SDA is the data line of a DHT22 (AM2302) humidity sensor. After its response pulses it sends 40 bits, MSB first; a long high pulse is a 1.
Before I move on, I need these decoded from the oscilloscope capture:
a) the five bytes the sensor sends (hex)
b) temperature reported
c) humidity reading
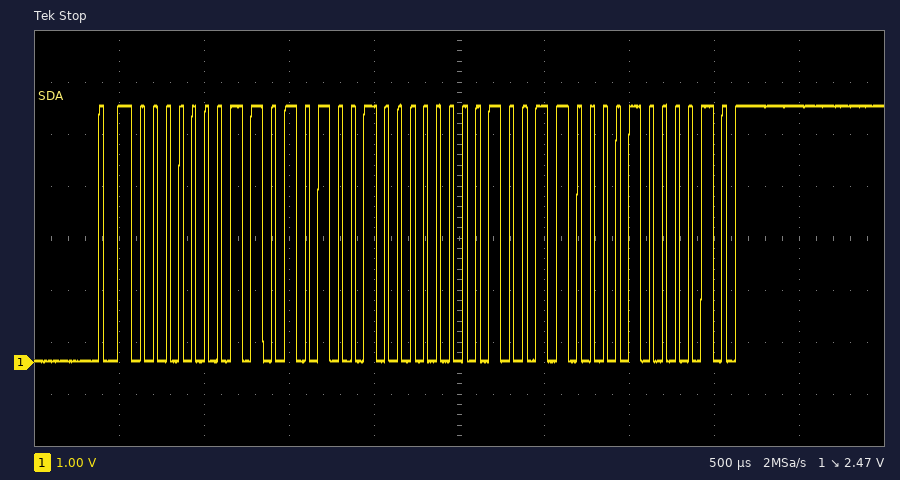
01 A9 00 98 42
15.2 °C
42.5 %
